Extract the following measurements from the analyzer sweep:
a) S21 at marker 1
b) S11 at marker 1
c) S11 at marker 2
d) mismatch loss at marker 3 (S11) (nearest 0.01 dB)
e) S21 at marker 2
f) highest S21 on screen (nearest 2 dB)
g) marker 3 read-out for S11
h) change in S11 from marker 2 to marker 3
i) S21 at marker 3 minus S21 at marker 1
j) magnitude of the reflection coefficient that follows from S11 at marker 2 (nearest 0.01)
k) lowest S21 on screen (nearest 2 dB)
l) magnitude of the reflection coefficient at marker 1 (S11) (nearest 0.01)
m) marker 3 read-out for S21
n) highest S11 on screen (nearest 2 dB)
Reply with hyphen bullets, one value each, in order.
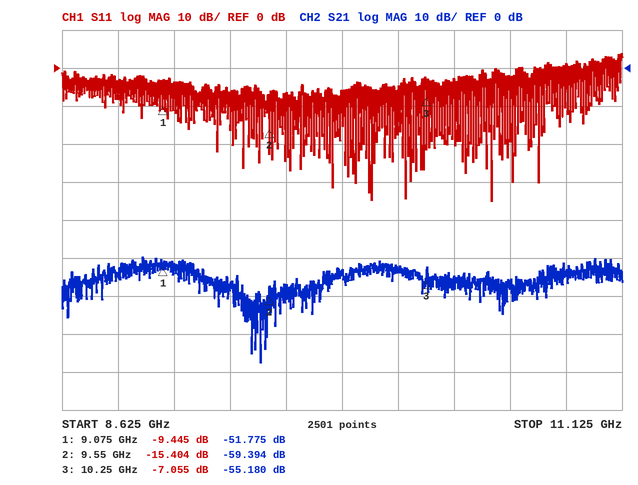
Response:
- -51.775 dB
- -9.445 dB
- -15.404 dB
- 0.95 dB
- -59.394 dB
- -50 dB
- -7.055 dB
- 8.349 dB
- -3.405 dB
- 0.17
- -78 dB
- 0.34
- -55.180 dB
- 4 dB
